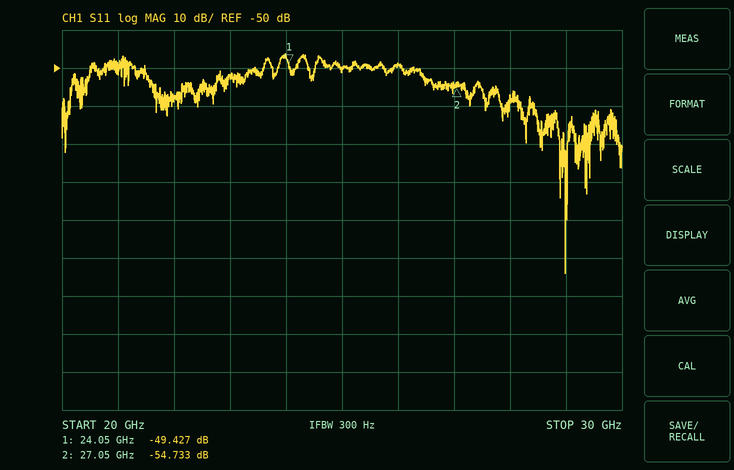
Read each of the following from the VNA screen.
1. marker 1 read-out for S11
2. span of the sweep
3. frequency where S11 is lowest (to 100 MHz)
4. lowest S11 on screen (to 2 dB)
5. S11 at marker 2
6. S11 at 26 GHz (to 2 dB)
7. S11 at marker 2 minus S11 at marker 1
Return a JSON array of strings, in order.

["-49.427 dB", "10 GHz", "29.0 GHz", "-104 dB", "-54.733 dB", "-50 dB", "-5.306 dB"]
